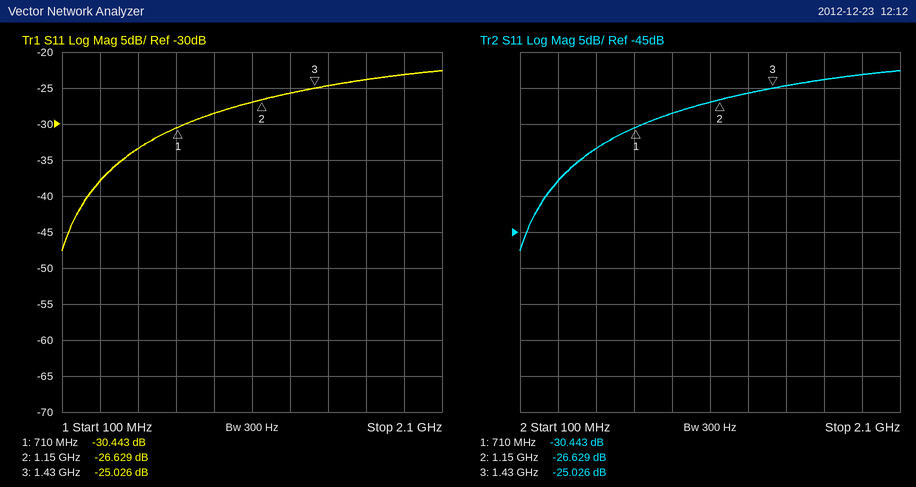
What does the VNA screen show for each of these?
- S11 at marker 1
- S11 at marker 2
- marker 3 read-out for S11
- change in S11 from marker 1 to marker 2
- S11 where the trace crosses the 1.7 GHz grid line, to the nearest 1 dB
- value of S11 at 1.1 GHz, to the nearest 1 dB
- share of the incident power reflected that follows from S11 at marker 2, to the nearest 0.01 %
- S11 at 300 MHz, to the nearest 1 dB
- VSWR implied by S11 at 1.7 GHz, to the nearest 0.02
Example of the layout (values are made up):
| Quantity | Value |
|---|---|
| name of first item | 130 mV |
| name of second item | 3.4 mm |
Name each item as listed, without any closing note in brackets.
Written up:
| Quantity | Value |
|---|---|
| S11 at marker 1 | -30.443 dB |
| S11 at marker 2 | -26.629 dB |
| marker 3 read-out for S11 | -25.026 dB |
| change in S11 from marker 1 to marker 2 | 3.814 dB |
| S11 where the trace crosses the 1.7 GHz grid line, to the nearest 1 dB | -24 dB |
| value of S11 at 1.1 GHz, to the nearest 1 dB | -27 dB |
| share of the incident power reflected that follows from S11 at marker 2, to the nearest 0.01 % | 0.22 % |
| S11 at 300 MHz, to the nearest 1 dB | -38 dB |
| VSWR implied by S11 at 1.7 GHz, to the nearest 0.02 | 1.14 |
